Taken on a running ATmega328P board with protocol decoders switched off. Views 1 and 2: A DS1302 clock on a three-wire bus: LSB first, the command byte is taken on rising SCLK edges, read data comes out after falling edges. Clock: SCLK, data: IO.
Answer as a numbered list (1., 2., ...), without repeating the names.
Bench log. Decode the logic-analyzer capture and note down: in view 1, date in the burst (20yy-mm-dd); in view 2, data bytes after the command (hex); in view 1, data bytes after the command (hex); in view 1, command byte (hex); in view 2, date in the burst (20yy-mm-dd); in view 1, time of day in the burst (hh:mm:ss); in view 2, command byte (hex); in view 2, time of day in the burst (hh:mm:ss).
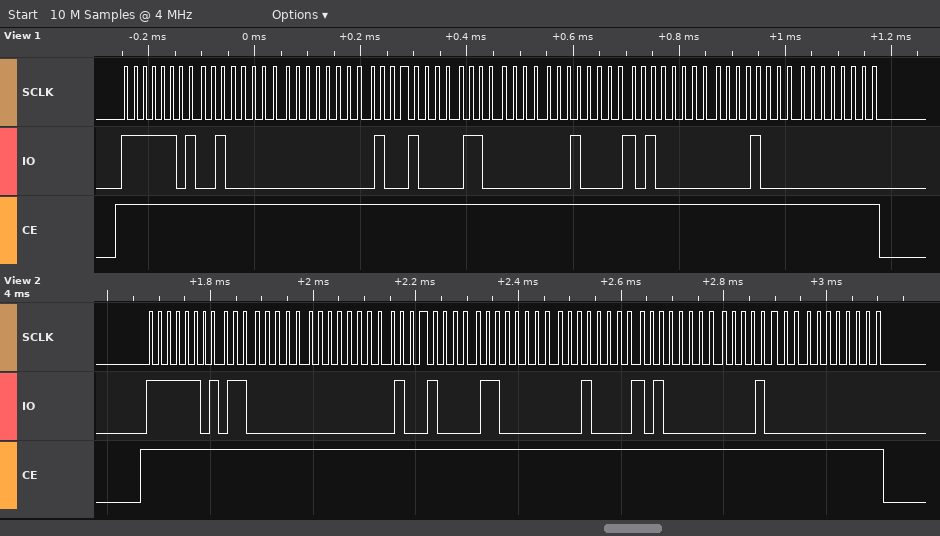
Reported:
1. 2010-08-06
2. 06 00 12 06 08 05 10 00
3. 04 00 12 06 08 05 10 00
4. 0xBF
5. 2010-08-06
6. 12:00:04
7. 0xBF
8. 12:00:06
